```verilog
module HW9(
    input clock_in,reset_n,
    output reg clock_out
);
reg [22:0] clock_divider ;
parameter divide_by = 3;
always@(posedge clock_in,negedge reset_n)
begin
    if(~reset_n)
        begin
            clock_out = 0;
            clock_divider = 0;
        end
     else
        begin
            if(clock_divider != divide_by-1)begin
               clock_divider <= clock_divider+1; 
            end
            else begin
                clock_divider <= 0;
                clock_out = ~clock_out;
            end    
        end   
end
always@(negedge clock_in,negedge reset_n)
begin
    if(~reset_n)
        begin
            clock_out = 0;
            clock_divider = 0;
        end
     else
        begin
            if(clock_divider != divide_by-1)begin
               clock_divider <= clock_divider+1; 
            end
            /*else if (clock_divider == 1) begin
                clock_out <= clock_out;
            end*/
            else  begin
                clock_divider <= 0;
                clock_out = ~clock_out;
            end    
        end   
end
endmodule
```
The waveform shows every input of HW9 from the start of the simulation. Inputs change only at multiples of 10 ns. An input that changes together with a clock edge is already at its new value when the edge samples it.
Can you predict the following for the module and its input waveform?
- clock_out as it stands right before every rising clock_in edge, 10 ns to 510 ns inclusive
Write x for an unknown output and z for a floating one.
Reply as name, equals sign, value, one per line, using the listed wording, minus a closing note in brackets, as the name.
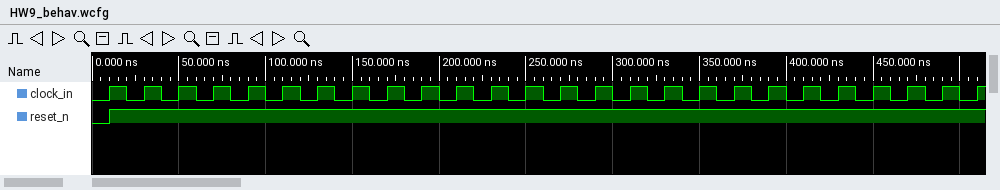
clock_out as it stands right before every rising clock_in edge, 10 ns to 510 ns inclusive = 0 0 1 0 0 1 0 0 1 0 0 1 0 0 1 0 0 1 0 0 1 0 0 1 0 0
